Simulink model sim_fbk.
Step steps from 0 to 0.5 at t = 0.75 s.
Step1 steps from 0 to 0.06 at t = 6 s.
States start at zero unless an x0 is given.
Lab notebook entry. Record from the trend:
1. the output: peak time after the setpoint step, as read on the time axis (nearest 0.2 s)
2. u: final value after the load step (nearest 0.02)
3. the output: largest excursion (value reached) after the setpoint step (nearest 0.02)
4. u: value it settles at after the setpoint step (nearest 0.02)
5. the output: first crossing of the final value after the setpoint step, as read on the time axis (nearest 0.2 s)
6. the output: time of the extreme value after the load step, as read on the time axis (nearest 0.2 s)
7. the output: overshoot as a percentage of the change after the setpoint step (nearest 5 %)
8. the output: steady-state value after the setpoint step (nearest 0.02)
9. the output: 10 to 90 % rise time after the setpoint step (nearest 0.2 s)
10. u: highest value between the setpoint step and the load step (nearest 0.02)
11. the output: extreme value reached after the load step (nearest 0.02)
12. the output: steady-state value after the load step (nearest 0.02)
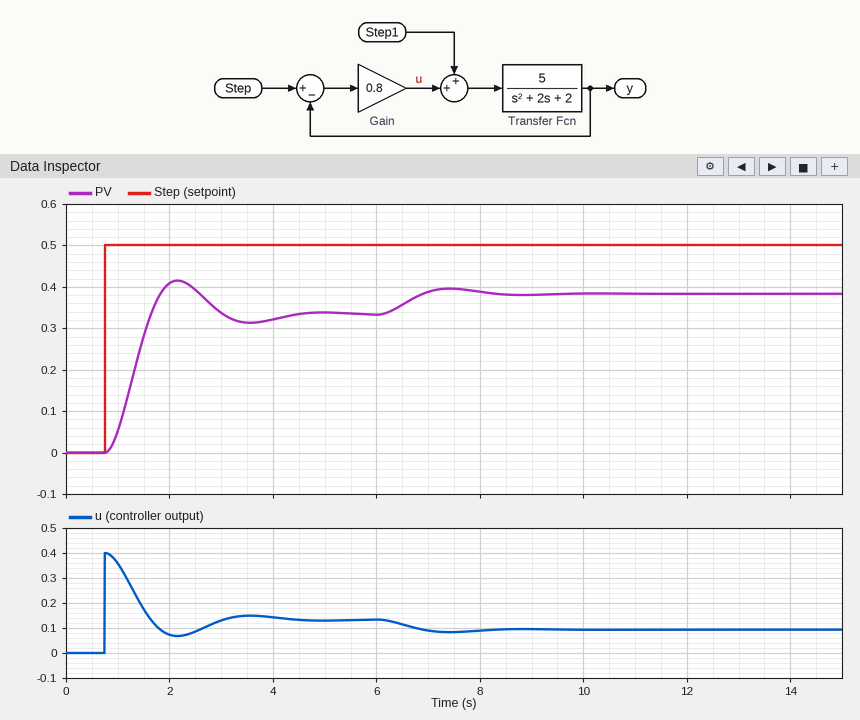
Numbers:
2.2 s
0.10
0.42
0.14
1.6 s
7.4 s
25 %
0.34
0.6 s
0.40
0.40
0.38
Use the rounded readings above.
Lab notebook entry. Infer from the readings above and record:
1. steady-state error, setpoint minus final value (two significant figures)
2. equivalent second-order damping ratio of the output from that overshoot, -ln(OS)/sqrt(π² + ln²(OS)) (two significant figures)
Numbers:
0.16
0.40
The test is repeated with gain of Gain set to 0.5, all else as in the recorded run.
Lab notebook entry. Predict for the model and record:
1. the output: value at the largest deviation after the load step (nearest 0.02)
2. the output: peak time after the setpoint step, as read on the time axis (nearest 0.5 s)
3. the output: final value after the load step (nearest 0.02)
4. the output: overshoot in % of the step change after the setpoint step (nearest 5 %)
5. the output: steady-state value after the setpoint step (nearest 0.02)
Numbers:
0.36
2.5 s
0.34
20 %
0.28
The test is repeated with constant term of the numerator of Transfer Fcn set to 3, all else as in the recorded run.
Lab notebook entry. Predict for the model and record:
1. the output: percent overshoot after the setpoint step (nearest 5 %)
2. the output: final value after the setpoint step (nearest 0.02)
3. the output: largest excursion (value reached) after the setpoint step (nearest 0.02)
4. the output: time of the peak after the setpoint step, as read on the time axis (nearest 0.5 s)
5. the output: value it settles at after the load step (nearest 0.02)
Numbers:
20 %
0.28
0.32
2.5 s
0.32
